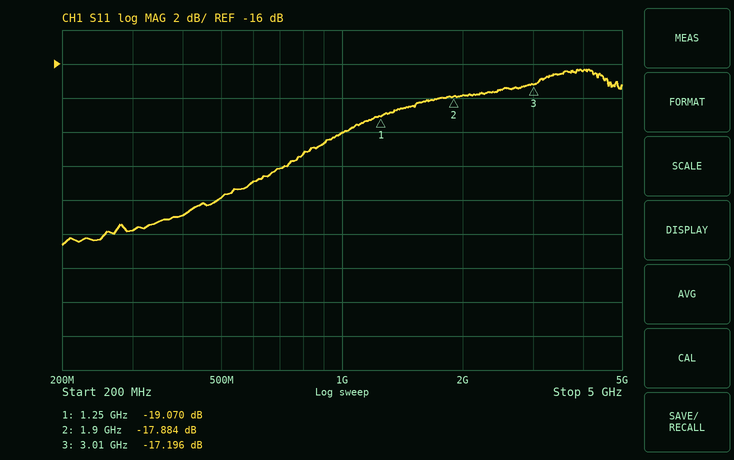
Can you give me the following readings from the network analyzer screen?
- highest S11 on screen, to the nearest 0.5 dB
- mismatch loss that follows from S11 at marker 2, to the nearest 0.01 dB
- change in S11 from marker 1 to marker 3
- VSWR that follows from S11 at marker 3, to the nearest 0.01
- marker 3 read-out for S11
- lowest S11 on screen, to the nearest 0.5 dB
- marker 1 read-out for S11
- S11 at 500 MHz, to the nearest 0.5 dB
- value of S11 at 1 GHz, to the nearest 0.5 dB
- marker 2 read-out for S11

-16.5 dB
0.07 dB
1.874 dB
1.32
-17.196 dB
-26.5 dB
-19.070 dB
-24.0 dB
-20.0 dB
-17.884 dB
